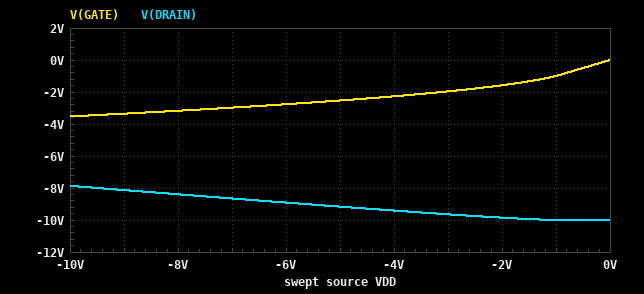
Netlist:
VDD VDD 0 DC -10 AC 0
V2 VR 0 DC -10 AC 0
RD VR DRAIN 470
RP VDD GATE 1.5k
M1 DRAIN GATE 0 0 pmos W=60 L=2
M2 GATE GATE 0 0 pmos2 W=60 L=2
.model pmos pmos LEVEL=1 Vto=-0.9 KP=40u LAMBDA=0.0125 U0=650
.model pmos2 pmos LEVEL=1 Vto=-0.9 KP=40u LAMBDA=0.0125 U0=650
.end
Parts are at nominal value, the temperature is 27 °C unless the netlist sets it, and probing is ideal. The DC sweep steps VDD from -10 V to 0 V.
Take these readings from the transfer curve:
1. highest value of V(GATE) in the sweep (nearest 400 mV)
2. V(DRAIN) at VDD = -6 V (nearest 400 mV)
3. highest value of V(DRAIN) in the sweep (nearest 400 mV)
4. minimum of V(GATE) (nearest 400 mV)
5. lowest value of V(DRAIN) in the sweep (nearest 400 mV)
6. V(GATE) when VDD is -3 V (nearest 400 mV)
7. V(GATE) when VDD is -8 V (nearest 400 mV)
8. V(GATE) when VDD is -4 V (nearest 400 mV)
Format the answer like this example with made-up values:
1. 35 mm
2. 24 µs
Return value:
1. 0 V
2. -8.8 V
3. -8.0 V
4. -3.6 V
5. -10.0 V
6. -2.0 V
7. -3.2 V
8. -2.4 V
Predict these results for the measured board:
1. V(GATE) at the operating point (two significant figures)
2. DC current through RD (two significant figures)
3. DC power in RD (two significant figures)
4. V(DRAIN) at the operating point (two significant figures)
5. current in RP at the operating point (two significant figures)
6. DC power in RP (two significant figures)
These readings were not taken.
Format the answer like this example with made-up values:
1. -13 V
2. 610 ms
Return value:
1. -3.5 V
2. 4.5 mA
3. 9.7 mW
4. -7.9 V
5. 4.3 mA
6. 28 mW
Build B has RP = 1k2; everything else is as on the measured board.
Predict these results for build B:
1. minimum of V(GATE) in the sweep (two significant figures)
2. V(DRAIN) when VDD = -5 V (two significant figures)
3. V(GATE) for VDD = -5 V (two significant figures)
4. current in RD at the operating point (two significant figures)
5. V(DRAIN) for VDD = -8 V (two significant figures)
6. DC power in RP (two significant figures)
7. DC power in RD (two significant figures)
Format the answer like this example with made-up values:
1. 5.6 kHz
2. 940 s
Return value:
1. -3.8 V
2. -9.0 V
3. -2.7 V
4. 5.4 mA
5. -8.1 V
6. 32 mW
7. 14 mW
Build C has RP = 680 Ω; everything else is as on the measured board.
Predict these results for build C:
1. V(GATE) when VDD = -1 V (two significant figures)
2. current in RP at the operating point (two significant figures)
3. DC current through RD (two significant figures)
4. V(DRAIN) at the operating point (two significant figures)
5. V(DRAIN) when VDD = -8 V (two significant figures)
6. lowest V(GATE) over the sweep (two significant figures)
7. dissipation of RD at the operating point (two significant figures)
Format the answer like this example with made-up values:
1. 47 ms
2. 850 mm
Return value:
1. -1.0 V
2. 8.1 mA
3. 8.3 mA
4. -6.1 V
5. -7.1 V
6. -4.5 V
7. 32 mW
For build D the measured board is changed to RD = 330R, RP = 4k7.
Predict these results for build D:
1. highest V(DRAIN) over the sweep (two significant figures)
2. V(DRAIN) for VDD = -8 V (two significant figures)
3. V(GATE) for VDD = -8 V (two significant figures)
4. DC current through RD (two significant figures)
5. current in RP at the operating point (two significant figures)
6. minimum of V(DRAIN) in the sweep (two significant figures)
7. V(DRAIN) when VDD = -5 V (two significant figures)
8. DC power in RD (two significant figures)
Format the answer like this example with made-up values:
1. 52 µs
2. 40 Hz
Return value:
1. -9.4 V
2. -9.6 V
3. -2.3 V
4. 1.7 mA
5. 1.6 mA
6. -10 V
7. -9.8 V
8. 990 µW
